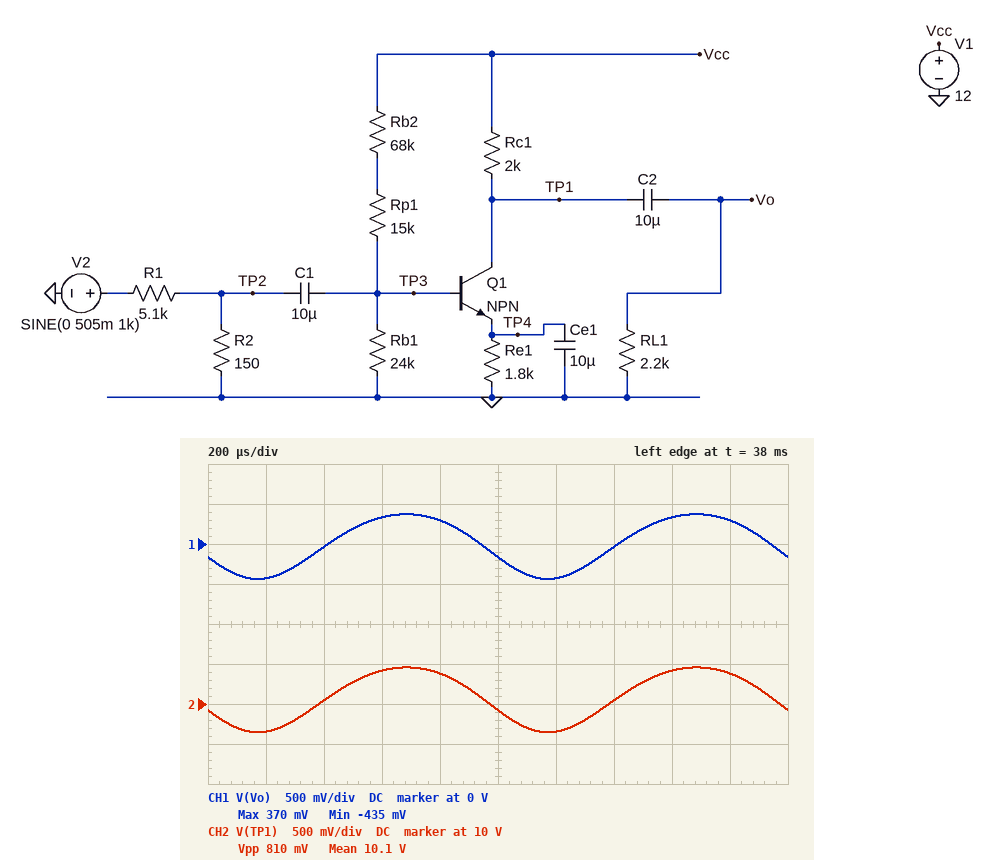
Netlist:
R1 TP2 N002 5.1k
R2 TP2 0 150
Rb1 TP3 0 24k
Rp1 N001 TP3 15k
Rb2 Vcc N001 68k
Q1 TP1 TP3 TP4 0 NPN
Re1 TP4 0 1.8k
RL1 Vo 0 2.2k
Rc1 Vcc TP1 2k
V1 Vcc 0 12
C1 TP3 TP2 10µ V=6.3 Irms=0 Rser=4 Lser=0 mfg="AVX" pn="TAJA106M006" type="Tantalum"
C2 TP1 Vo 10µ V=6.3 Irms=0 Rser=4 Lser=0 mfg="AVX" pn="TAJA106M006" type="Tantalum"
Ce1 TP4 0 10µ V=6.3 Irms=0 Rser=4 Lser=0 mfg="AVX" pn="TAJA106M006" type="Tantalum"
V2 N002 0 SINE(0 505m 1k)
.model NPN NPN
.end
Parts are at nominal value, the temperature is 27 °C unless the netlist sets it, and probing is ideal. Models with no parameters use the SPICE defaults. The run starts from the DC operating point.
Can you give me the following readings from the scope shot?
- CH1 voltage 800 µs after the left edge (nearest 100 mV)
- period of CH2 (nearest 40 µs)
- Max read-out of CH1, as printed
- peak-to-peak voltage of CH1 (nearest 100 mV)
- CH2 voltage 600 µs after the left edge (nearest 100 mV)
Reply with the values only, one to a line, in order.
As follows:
300 mV
1.00 ms
370 mV
800 mV
10.4 V
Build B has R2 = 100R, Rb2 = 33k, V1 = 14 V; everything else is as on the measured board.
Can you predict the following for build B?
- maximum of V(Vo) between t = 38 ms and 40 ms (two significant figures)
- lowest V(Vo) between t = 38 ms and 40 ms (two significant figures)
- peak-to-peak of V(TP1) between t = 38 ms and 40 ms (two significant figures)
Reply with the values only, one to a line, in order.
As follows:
400 mV
-420 mV
820 mV
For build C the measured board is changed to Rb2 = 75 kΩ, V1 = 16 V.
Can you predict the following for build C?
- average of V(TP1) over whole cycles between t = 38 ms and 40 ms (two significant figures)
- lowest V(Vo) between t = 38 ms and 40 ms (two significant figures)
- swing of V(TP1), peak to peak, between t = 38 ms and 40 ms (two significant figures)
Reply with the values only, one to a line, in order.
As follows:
13 V
-520 mV
980 mV
